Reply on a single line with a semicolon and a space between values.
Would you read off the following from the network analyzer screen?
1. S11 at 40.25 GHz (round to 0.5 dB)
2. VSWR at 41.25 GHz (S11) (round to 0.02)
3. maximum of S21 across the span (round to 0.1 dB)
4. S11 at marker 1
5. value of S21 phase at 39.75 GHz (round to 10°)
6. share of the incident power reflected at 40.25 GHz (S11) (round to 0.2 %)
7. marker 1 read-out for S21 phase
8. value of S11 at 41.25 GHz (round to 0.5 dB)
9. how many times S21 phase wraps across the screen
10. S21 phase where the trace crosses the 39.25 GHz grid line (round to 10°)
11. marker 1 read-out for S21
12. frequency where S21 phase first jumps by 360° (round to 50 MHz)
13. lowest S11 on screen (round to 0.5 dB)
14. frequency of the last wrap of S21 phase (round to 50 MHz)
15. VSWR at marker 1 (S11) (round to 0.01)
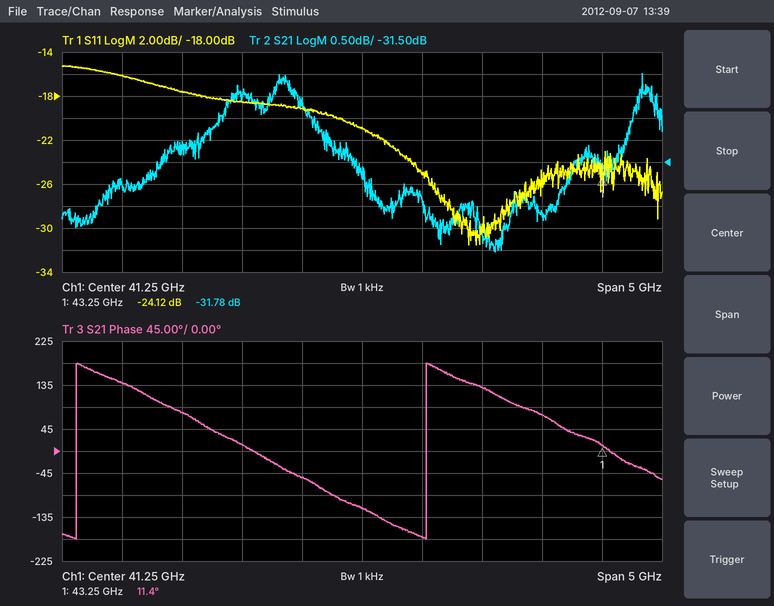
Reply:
-18.5 dB; 1.20; -29.5 dB; -24.12 dB; 80°; 1.4 %; 11.4°; -21.0 dB; 2; 140°; -31.78 dB; 38.85 GHz; -31.5 dB; 41.80 GHz; 1.13
